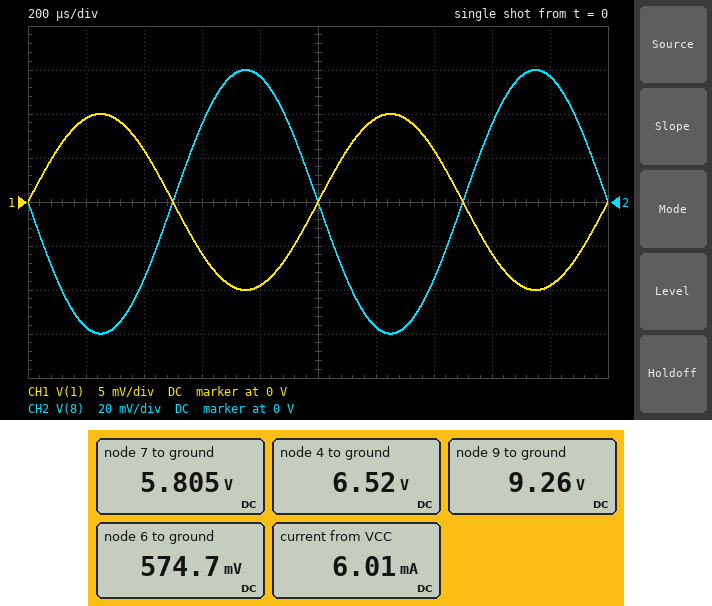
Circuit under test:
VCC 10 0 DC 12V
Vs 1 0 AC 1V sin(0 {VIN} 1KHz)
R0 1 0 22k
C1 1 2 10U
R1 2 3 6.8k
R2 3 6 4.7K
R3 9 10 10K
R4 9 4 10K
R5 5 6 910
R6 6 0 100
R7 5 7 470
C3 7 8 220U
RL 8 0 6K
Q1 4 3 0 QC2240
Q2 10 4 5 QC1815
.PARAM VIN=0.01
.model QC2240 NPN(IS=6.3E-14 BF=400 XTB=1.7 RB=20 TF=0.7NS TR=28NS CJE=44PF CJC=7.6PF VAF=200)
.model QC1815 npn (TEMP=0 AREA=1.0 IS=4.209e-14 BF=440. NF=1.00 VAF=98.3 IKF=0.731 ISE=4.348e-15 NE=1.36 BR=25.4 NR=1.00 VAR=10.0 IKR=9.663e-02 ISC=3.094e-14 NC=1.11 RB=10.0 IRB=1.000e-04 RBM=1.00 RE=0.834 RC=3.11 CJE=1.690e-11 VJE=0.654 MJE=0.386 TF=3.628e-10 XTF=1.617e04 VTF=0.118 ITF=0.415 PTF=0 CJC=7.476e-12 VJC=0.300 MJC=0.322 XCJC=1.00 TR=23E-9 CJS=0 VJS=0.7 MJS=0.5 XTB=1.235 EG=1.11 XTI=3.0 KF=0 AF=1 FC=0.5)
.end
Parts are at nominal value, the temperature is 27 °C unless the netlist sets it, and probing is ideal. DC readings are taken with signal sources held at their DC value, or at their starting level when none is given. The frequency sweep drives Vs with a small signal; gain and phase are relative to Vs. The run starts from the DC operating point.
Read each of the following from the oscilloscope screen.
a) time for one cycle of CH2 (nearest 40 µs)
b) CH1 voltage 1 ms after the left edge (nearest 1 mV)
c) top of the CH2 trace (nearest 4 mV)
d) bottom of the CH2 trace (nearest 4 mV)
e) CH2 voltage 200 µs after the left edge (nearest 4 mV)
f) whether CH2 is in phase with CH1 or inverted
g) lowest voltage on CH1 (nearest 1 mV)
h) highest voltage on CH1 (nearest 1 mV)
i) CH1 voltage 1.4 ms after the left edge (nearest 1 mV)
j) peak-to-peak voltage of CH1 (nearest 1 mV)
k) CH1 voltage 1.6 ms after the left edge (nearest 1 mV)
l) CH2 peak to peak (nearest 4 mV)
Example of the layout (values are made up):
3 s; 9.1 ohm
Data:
1.00 ms; 0 V; 60 mV; -60 mV; -56 mV; inverted; -10 mV; 10 mV; 6 mV; 20 mV; -6 mV; 120 mV
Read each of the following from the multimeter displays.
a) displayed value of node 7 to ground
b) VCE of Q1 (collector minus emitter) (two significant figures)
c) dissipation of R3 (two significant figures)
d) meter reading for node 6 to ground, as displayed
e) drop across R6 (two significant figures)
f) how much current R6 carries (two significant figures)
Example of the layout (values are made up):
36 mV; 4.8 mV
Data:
5.805 V; 6.5 V; 750 µW; 574.7 mV; 570 mV; 5.7 mA
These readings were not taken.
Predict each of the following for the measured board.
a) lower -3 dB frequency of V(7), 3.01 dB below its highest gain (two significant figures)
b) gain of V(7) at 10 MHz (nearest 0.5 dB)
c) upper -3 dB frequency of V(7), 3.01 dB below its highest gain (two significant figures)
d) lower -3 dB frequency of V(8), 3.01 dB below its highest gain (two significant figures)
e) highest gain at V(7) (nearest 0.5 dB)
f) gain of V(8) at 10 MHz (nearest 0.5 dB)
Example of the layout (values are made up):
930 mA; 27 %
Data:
2.3 Hz; -8.0 dB; 870 kHz; 2.3 Hz; 15.5 dB; -8.0 dB
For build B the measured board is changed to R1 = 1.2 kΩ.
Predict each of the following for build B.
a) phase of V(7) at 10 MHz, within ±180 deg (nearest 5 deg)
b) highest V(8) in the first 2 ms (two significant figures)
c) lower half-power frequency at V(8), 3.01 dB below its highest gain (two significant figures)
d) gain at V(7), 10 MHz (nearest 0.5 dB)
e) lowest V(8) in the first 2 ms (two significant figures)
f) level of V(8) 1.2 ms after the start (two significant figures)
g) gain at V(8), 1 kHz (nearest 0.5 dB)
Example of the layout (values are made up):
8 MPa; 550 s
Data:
60 deg; 290 mV; 11 Hz; 6.5 dB; -290 mV; -280 mV; 29.5 dB
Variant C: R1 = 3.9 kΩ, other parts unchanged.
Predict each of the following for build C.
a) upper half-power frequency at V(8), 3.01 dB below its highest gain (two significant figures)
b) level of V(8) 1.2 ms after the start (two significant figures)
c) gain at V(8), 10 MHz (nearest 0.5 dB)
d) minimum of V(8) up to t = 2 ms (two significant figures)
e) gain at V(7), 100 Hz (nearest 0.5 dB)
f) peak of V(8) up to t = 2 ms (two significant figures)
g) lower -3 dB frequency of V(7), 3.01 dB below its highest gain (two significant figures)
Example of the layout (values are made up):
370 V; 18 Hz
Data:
880 kHz; -97 mV; -3.0 dB; -100 mV; 20.0 dB; 100 mV; 3.8 Hz
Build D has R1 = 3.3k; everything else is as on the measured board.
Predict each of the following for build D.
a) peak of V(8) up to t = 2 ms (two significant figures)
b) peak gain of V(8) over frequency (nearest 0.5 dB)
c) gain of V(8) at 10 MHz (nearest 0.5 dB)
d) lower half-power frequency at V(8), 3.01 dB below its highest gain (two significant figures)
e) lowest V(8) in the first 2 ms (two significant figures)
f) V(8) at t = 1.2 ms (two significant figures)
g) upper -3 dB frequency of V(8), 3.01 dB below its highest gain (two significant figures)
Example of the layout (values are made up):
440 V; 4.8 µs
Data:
120 mV; 21.5 dB; -1.5 dB; 4.5 Hz; -120 mV; -110 mV; 880 kHz
